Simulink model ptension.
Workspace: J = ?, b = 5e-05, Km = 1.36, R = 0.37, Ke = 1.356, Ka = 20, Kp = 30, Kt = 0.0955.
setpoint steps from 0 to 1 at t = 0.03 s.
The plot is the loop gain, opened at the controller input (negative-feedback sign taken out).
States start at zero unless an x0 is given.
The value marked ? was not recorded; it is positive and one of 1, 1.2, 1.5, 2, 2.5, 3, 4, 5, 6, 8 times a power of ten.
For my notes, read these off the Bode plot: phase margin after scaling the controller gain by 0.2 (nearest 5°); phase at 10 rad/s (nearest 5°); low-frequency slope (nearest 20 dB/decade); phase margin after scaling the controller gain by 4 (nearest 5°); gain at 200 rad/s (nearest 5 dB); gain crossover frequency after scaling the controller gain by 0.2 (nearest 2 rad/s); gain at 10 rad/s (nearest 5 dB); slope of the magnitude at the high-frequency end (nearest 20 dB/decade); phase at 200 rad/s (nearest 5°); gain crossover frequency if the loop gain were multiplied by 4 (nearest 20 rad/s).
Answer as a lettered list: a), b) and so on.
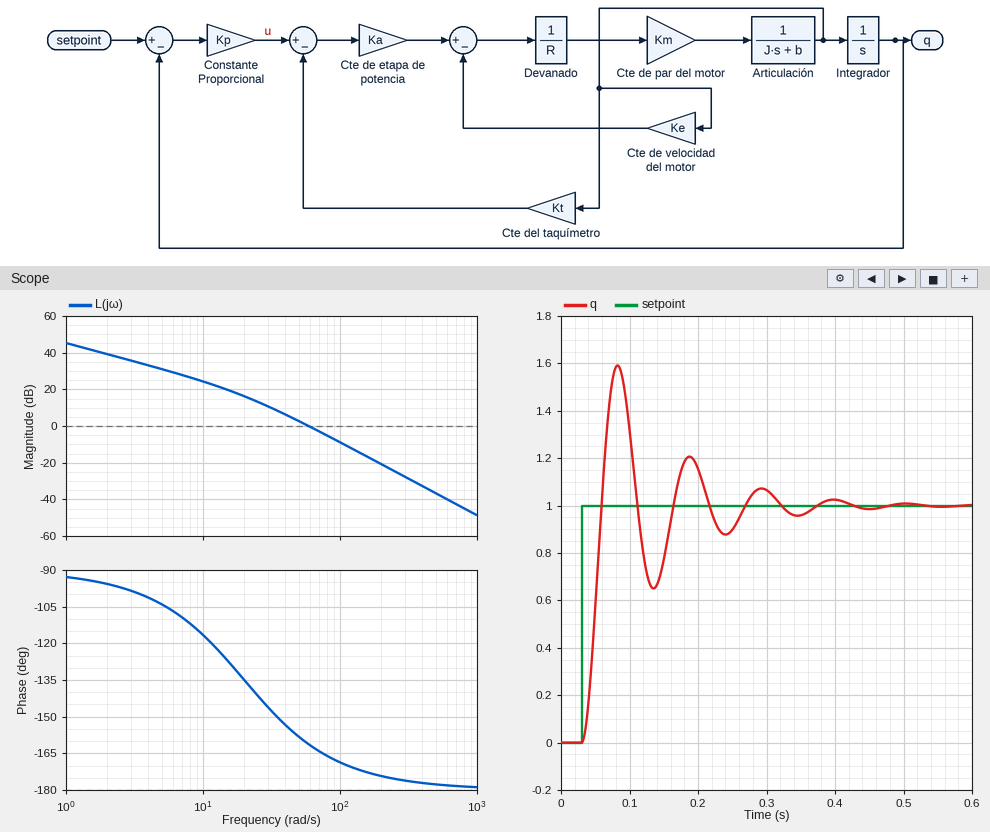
a) 40°
b) -115°
c) -20 dB/decade
d) 10°
e) -20 dB
f) 24 rad/s
g) 25 dB
h) -40 dB/decade
i) -175°
j) 120 rad/s
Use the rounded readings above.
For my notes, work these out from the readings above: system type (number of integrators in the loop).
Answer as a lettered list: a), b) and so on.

a) 1
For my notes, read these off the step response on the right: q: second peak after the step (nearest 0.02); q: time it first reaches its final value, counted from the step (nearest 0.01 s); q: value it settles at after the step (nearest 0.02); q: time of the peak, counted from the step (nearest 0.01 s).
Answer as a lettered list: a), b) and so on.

a) 1.20
b) 0.03 s
c) 1.00
d) 0.05 s
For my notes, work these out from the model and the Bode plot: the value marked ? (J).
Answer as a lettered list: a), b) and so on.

a) 0.6
